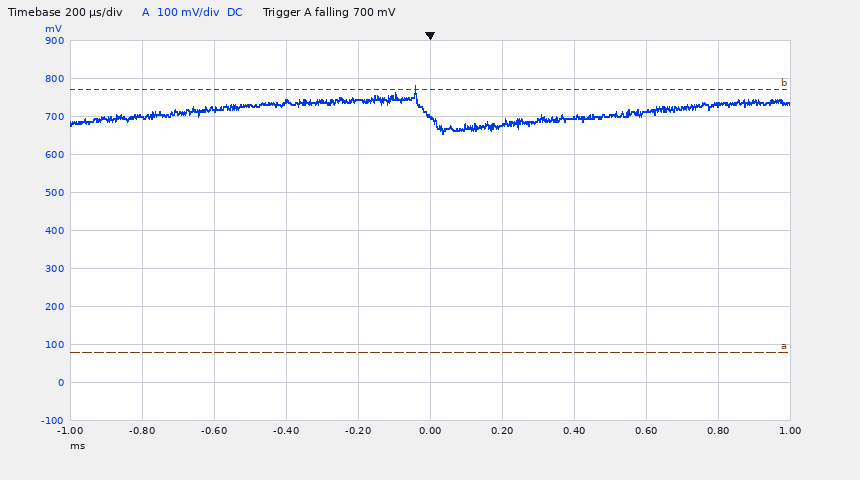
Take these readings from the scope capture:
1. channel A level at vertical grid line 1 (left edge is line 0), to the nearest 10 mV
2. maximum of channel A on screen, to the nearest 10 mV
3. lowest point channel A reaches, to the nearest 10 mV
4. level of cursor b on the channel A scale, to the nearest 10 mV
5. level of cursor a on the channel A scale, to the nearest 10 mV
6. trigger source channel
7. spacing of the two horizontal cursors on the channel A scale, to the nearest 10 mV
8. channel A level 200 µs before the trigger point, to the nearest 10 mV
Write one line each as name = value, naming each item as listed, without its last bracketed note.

channel A level at vertical grid line 1 (left edge is line 0), to the nearest 10 mV = 700 mV
maximum of channel A on screen, to the nearest 10 mV = 780 mV
lowest point channel A reaches, to the nearest 10 mV = 660 mV
level of cursor b on the channel A scale, to the nearest 10 mV = 770 mV
level of cursor a on the channel A scale, to the nearest 10 mV = 80 mV
trigger source channel = channel A
spacing of the two horizontal cursors on the channel A scale, to the nearest 10 mV = 690 mV
channel A level 200 µs before the trigger point, to the nearest 10 mV = 740 mV
